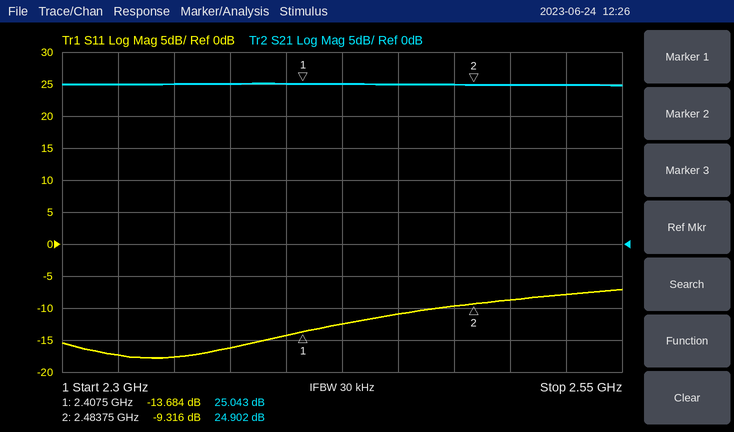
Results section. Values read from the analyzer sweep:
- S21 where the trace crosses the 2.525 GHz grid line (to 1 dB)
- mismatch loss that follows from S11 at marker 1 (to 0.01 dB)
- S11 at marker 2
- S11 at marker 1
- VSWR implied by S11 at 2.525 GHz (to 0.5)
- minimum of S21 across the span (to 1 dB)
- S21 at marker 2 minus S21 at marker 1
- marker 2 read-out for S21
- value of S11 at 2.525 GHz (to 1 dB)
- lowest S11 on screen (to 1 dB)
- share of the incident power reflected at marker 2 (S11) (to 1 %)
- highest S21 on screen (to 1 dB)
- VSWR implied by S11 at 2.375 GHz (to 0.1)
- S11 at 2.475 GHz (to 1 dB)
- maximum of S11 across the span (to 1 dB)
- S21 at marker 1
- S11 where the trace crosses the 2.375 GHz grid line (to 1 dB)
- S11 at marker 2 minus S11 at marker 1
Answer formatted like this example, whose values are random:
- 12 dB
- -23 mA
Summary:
- 25 dB
- 0.19 dB
- -9.316 dB
- -13.684 dB
- 2.5
- 25 dB
- -0.141 dB
- 24.902 dB
- -8 dB
- -18 dB
- 12 %
- 25 dB
- 1.4
- -10 dB
- -7 dB
- 25.043 dB
- -16 dB
- 4.368 dB
